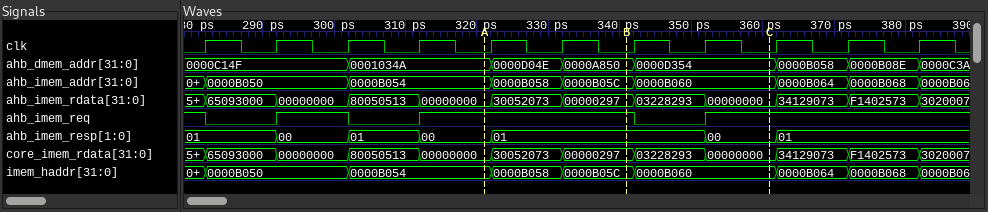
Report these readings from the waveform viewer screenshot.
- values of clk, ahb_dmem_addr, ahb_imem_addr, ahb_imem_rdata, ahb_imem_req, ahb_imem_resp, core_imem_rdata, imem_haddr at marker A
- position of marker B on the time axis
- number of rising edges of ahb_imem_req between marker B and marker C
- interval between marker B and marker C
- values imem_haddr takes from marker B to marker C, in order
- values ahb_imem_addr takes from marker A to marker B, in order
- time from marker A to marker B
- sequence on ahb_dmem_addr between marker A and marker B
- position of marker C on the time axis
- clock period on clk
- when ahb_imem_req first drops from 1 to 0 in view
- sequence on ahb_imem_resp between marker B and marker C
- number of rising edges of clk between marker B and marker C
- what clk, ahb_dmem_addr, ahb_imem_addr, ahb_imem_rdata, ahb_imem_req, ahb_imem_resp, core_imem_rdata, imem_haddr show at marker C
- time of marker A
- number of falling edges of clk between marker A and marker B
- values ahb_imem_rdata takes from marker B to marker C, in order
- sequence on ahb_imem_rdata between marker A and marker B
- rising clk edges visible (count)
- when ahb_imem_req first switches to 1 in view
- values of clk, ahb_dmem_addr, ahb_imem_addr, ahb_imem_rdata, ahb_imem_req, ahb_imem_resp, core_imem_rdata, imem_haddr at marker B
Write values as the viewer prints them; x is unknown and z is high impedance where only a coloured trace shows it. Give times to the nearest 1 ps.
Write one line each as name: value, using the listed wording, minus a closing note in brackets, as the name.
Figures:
values of clk, ahb_dmem_addr, ahb_imem_addr, ahb_imem_rdata, ahb_imem_req, ahb_imem_resp, core_imem_rdata, imem_haddr at marker A: clk=0, ahb_dmem_addr=0001034A, ahb_imem_addr=0000B054, ahb_imem_rdata=00000000, ahb_imem_req=1, ahb_imem_resp=00, core_imem_rdata=00000000, imem_haddr=0000B054
position of marker B on the time axis: 341 ps
number of rising edges of ahb_imem_req between marker B and marker C: 1
interval between marker B and marker C: 20 ps
values imem_haddr takes from marker B to marker C, in order: 0000B05C, 0000B060
values ahb_imem_addr takes from marker A to marker B, in order: 0000B054, 0000B058, 0000B05C
time from marker A to marker B: 20 ps
sequence on ahb_dmem_addr between marker A and marker B: 0001034A, 0000D04E, 0000A850
position of marker C on the time axis: 361 ps
clock period on clk: 10 ps
when ahb_imem_req first drops from 1 to 0 in view: 282 ps
sequence on ahb_imem_resp between marker B and marker C: 01, 00
number of rising edges of clk between marker B and marker C: 2
what clk, ahb_dmem_addr, ahb_imem_addr, ahb_imem_rdata, ahb_imem_req, ahb_imem_resp, core_imem_rdata, imem_haddr show at marker C: clk=0, ahb_dmem_addr=0000D354, ahb_imem_addr=0000B060, ahb_imem_rdata=00000000, ahb_imem_req=1, ahb_imem_resp=00, core_imem_rdata=00000000, imem_haddr=0000B060
time of marker A: 321 ps
number of falling edges of clk between marker A and marker B: 2
values ahb_imem_rdata takes from marker B to marker C, in order: 00000297, 03228293, 00000000
sequence on ahb_imem_rdata between marker A and marker B: 00000000, 30052073, 00000297
rising clk edges visible: 11
when ahb_imem_req first switches to 1 in view: 292 ps
values of clk, ahb_dmem_addr, ahb_imem_addr, ahb_imem_rdata, ahb_imem_req, ahb_imem_resp, core_imem_rdata, imem_haddr at marker B: clk=0, ahb_dmem_addr=0000A850, ahb_imem_addr=0000B05C, ahb_imem_rdata=00000297, ahb_imem_req=1, ahb_imem_resp=01, core_imem_rdata=00000297, imem_haddr=0000B05C
